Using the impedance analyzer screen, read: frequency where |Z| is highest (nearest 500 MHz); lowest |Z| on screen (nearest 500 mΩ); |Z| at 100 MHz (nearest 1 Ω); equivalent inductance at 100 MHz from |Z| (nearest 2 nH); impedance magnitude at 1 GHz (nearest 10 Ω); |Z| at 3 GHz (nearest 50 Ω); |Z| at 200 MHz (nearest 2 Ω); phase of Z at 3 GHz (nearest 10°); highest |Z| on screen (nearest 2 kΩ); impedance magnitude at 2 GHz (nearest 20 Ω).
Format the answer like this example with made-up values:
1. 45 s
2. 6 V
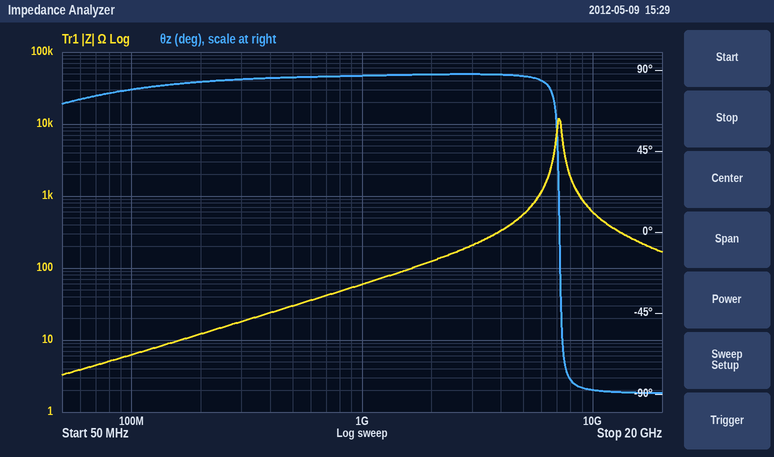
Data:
1. 7.0 GHz
2. 3.5 Ω
3. 6 Ω
4. 10 nH
5. 60 Ω
6. 200 Ω
7. 12 Ω
8. 90°
9. 12 kΩ
10. 120 Ω
